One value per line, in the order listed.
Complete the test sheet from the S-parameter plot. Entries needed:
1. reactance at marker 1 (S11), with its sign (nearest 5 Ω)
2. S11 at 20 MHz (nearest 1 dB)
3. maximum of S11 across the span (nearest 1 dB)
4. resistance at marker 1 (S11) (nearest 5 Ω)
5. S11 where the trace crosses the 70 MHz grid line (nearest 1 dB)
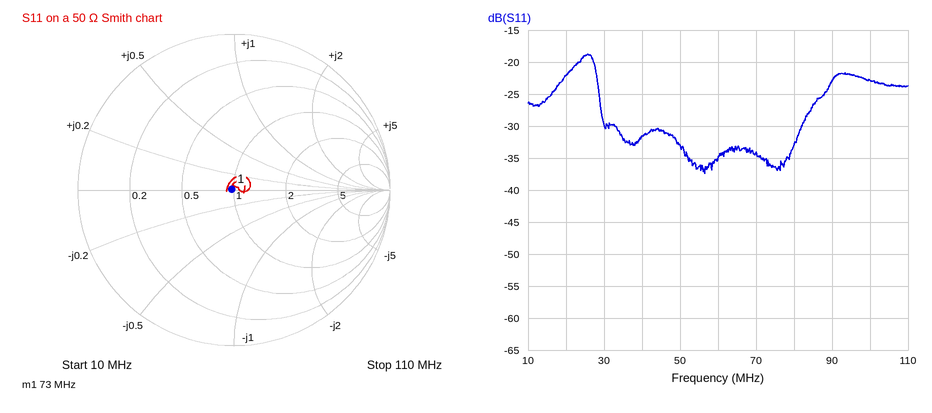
0 Ω
-22 dB
-19 dB
50 Ω
-34 dB
